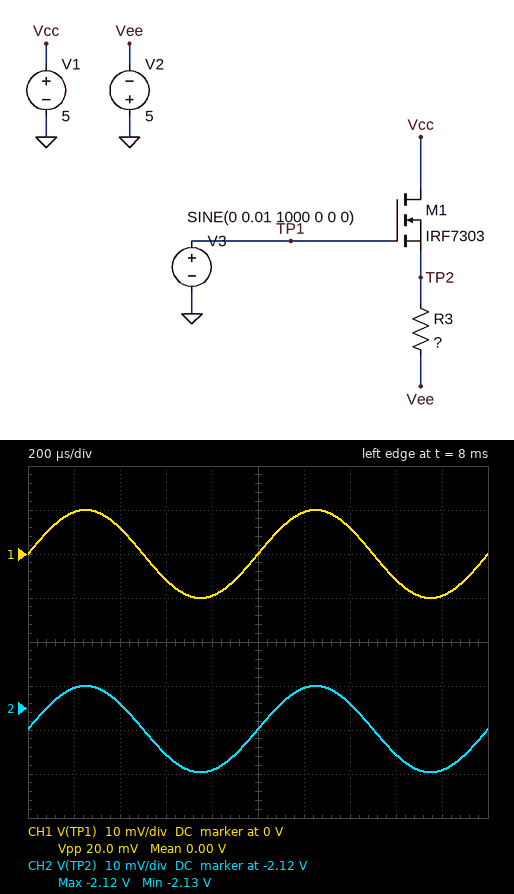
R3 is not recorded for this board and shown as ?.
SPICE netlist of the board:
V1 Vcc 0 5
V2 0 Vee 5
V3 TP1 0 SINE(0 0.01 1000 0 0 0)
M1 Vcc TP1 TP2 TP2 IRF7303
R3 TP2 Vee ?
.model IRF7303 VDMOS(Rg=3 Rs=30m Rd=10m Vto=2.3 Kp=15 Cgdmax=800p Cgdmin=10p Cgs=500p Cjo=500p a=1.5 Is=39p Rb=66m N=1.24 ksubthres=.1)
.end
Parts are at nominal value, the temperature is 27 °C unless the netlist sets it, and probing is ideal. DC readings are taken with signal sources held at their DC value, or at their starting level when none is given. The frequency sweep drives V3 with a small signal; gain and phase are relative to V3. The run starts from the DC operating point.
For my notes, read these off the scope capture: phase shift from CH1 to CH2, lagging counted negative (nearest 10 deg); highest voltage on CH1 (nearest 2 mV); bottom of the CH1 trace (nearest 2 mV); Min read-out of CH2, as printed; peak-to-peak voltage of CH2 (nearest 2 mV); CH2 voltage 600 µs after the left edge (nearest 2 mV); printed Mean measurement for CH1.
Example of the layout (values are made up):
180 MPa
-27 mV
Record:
0 deg
10 mV
-10 mV
-2.13 V
20 mV
-2.130 V
0.00 V
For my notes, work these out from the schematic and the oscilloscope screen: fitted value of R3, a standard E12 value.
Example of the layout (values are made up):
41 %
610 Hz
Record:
1.5 kΩ
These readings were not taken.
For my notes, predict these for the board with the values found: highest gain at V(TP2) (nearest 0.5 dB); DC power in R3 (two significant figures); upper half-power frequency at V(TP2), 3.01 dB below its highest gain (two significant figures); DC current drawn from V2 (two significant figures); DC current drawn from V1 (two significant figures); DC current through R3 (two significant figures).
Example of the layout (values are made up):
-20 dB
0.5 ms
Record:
0 dB
5.5 mW
150 MHz
1.9 mA
1.9 mA
1.9 mA
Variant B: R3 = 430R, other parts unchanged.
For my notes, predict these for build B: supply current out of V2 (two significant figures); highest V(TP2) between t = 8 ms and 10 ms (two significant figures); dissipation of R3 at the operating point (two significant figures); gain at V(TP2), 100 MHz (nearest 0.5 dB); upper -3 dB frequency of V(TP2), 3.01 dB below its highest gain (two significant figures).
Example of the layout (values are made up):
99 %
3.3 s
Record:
6.5 mA
-2.2 V
18 mW
-2.0 dB
180 MHz
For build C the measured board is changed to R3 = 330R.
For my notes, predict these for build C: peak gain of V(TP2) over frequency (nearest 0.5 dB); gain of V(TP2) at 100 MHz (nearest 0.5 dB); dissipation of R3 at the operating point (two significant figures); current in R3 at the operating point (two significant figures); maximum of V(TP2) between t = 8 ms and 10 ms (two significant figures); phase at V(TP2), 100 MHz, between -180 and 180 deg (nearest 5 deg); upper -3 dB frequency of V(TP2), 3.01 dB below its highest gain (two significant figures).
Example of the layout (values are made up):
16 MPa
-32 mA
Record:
0 dB
-2.0 dB
24 mW
8.5 mA
-2.2 V
-25 deg
190 MHz
